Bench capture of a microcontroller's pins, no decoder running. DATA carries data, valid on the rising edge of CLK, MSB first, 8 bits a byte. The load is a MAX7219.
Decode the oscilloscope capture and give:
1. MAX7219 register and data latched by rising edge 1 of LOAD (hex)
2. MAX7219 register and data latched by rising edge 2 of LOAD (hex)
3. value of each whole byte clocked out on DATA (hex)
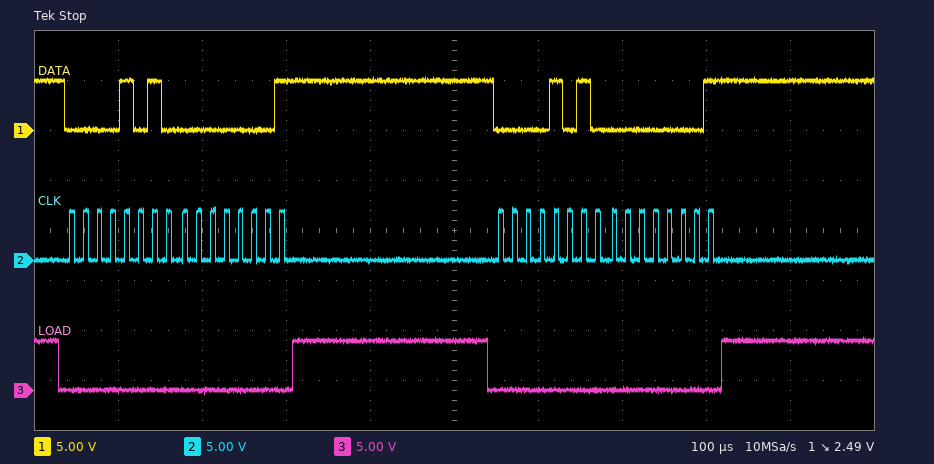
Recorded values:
register 0xA, data 0x01
register 0xA, data 0x01
0x0A 0x01 0x0A 0x01
